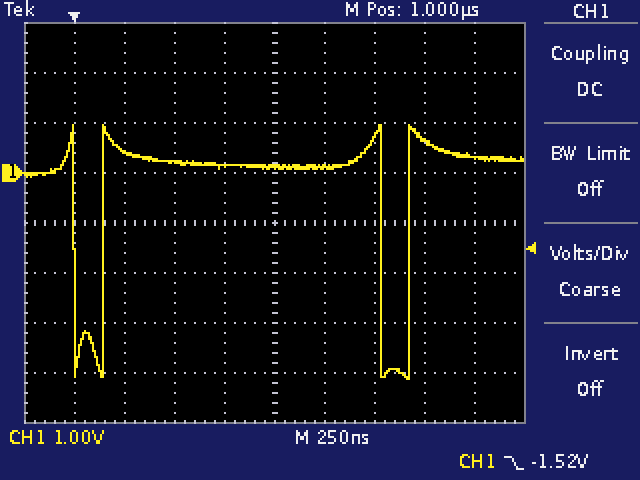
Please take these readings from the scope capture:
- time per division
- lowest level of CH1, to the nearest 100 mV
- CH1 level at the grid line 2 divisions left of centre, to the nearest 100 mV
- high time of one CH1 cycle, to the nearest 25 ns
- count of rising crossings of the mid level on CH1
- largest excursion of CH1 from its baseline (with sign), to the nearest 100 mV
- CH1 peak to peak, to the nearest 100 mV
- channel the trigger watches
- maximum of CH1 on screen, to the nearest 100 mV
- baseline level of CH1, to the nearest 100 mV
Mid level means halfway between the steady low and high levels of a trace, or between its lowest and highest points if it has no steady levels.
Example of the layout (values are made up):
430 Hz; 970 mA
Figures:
250 ns; -4.1 V; 200 mV; 1.400 µs; 2; -4.3 V; 5.1 V; CH1; 1.0 V; 200 mV
